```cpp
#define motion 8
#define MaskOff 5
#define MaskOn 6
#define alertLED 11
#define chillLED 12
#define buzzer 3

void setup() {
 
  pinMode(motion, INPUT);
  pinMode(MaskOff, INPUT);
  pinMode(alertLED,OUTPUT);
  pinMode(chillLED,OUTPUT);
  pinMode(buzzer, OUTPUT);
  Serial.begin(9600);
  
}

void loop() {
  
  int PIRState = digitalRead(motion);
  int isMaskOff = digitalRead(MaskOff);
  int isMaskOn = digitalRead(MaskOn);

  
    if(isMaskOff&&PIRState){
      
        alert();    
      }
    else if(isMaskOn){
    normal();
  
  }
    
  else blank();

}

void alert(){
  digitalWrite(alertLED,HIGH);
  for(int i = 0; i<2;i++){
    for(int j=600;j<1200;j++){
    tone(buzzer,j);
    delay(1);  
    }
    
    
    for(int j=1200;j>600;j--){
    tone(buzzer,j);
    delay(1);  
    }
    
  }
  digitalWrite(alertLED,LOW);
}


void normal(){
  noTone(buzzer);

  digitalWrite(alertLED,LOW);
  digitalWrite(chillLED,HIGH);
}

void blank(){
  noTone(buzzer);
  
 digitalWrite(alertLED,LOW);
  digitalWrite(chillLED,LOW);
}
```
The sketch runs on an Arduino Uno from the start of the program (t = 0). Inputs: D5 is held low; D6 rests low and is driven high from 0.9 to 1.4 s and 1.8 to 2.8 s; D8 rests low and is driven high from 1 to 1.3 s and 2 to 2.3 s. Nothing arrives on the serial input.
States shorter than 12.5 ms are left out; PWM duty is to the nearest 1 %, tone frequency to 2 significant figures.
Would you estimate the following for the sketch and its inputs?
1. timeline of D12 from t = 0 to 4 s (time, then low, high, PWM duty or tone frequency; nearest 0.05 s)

0 s low; 0.9 s high; 1.4 s low; 1.8 s high; 2.8 s low
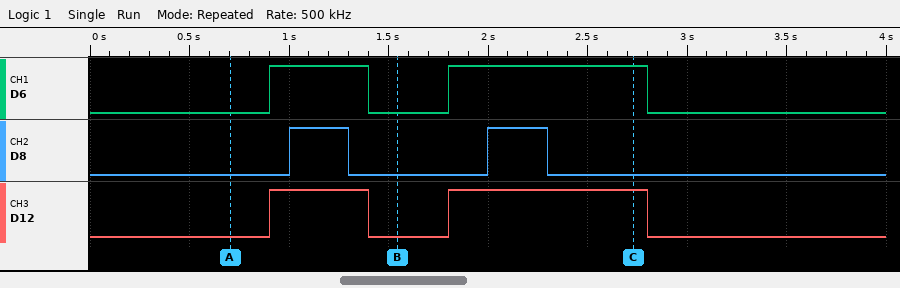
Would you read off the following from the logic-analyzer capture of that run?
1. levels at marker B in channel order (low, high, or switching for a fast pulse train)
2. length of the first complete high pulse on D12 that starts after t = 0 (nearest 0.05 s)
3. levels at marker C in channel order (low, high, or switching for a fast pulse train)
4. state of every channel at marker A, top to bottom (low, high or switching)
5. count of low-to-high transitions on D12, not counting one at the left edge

D6 low, D8 low, D12 low
0.50 s
D6 high, D8 low, D12 high
D6 low, D8 low, D12 low
2
